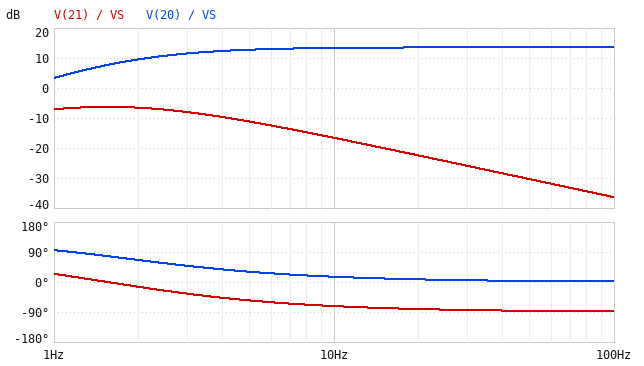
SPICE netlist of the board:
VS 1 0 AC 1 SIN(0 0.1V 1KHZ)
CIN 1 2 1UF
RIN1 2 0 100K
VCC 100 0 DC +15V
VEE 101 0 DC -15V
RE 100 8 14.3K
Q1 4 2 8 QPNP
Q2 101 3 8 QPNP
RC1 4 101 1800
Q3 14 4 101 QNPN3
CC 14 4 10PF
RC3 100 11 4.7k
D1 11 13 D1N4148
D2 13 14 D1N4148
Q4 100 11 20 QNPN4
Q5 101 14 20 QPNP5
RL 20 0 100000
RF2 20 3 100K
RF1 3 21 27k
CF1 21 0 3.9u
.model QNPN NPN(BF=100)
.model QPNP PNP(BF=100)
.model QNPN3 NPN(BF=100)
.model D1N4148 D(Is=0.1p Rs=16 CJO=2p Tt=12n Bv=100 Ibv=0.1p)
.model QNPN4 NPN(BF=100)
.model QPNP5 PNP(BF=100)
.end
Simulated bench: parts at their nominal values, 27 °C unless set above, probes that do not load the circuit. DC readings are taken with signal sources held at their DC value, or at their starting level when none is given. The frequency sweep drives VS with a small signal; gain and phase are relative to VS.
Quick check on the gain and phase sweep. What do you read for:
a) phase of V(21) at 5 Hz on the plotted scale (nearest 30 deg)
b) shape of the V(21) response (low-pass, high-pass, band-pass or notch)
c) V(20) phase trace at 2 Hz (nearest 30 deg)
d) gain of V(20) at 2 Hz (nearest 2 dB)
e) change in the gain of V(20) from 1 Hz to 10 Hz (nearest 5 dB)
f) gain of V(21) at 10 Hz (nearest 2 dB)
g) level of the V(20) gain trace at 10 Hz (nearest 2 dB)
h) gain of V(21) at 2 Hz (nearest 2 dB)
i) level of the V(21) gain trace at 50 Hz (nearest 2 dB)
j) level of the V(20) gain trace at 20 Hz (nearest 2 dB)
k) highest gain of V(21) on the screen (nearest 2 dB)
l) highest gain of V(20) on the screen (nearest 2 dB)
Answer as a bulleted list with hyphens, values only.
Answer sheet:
- -60 deg
- low-pass
- 60 deg
- 10 dB
- 10 dB
- -16 dB
- 14 dB
- -6 dB
- -30 dB
- 14 dB
- -6 dB
- 14 dB
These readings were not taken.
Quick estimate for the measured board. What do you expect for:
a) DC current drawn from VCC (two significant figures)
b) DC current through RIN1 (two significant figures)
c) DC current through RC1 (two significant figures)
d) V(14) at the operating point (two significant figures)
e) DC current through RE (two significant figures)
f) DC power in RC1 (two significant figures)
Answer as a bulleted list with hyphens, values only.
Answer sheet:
- 4.0 mA
- 4.8 µA
- 450 µA
- -680 mV
- 960 µA
- 360 µW
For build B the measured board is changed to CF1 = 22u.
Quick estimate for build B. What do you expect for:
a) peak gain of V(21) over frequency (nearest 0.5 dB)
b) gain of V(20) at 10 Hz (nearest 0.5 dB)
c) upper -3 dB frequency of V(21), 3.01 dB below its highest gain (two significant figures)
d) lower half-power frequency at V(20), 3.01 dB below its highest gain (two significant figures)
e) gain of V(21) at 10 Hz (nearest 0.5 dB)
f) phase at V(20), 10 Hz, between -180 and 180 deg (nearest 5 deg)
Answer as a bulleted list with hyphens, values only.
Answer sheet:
- -17.0 dB
- 13.5 dB
- 2.1 Hz
- 1.7 Hz
- -31.5 dB
- 10 deg
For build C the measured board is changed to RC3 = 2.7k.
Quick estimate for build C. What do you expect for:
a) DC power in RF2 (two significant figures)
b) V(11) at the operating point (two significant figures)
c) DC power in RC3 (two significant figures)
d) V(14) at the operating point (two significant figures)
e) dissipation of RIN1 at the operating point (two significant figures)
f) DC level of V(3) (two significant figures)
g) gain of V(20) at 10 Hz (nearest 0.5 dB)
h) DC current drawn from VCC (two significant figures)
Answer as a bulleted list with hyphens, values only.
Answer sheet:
- 2.0 µW
- 790 mV
- 75 mW
- -660 mV
- 2.6 µW
- 510 mV
- 13.5 dB
- 6.4 mA
